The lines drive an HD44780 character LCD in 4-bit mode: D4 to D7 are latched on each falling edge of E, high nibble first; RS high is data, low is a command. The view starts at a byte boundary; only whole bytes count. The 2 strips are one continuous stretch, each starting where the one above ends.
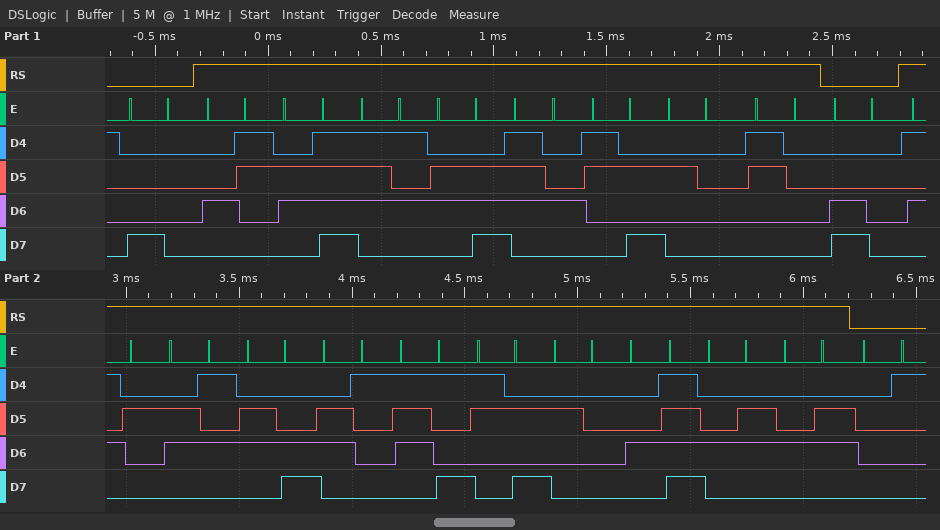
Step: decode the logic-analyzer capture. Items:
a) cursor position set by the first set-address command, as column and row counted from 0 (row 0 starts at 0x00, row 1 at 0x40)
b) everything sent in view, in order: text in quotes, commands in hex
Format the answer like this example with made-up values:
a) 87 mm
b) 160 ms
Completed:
a) column 0, row 0
b) 0x80 "Count: 0" 0xC0 "Relay: OFF" 0x01
